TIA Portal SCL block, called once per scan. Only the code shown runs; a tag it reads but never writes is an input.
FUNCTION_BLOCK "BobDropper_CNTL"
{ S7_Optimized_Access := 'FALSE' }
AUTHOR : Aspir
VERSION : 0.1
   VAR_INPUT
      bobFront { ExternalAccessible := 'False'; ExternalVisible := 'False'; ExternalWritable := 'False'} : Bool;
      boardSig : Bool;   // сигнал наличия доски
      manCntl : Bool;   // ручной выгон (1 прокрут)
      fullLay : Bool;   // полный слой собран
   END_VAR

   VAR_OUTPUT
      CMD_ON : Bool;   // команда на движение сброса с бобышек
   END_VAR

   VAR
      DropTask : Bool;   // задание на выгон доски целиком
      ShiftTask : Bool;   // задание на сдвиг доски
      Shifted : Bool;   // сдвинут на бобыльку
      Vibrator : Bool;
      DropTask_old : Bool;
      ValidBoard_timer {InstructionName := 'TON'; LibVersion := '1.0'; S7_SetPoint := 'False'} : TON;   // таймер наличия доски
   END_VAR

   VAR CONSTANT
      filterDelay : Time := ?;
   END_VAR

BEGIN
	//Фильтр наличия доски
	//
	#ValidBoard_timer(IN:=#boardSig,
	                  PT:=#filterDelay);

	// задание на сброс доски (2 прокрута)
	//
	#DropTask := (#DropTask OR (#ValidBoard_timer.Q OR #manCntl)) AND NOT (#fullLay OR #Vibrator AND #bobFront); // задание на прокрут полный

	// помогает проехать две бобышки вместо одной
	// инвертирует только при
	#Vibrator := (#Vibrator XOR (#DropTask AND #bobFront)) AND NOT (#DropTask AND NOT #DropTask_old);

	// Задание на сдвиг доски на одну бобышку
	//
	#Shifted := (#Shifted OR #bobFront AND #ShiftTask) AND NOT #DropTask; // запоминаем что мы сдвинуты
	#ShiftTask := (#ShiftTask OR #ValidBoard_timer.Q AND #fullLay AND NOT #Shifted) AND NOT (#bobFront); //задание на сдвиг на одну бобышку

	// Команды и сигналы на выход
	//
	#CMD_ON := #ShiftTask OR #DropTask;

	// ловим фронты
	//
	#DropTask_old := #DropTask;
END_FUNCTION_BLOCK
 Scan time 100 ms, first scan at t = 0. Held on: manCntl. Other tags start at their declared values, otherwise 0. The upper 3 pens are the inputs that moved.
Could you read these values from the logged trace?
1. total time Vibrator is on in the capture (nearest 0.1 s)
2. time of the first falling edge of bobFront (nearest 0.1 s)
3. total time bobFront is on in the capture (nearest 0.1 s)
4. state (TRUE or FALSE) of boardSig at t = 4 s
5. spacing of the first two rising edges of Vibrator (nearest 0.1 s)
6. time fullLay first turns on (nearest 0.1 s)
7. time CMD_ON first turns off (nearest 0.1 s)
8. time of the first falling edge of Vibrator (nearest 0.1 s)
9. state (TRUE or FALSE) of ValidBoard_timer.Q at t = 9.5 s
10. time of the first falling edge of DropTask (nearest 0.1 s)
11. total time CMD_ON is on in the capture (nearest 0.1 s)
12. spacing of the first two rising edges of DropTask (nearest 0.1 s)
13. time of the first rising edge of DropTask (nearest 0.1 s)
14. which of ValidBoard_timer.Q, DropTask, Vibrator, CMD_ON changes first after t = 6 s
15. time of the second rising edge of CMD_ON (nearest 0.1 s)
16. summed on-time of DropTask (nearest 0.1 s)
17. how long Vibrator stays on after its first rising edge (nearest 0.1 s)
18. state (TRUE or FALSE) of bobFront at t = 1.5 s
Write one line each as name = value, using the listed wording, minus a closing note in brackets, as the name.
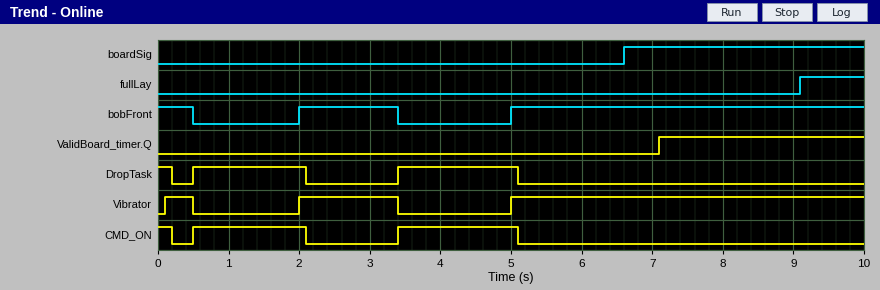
total time Vibrator is on in the capture = 6.8 s
time of the first falling edge of bobFront = 0.5 s
total time bobFront is on in the capture = 6.9 s
state (TRUE or FALSE) of boardSig at t = 4 s = FALSE
spacing of the first two rising edges of Vibrator = 1.9 s
time fullLay first turns on = 9.1 s
time CMD_ON first turns off = 0.2 s
time of the first falling edge of Vibrator = 0.5 s
state (TRUE or FALSE) of ValidBoard_timer.Q at t = 9.5 s = TRUE
time of the first falling edge of DropTask = 0.2 s
total time CMD_ON is on in the capture = 3.5 s
spacing of the first two rising edges of DropTask = 2.9 s
time of the first rising edge of DropTask = 0.5 s
which of ValidBoard_timer.Q, DropTask, Vibrator, CMD_ON changes first after t = 6 s = ValidBoard_timer.Q
time of the second rising edge of CMD_ON = 3.4 s
summed on-time of DropTask = 3.5 s
how long Vibrator stays on after its first rising edge = 0.4 s
state (TRUE or FALSE) of bobFront at t = 1.5 s = FALSE
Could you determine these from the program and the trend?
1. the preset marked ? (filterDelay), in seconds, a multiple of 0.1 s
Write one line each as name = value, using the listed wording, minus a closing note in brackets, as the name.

the preset marked ? (filterDelay), in seconds, a multiple of 0.1 s = 0.5 s
